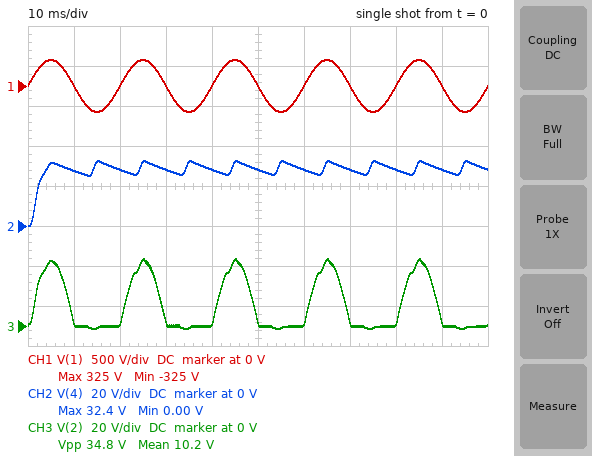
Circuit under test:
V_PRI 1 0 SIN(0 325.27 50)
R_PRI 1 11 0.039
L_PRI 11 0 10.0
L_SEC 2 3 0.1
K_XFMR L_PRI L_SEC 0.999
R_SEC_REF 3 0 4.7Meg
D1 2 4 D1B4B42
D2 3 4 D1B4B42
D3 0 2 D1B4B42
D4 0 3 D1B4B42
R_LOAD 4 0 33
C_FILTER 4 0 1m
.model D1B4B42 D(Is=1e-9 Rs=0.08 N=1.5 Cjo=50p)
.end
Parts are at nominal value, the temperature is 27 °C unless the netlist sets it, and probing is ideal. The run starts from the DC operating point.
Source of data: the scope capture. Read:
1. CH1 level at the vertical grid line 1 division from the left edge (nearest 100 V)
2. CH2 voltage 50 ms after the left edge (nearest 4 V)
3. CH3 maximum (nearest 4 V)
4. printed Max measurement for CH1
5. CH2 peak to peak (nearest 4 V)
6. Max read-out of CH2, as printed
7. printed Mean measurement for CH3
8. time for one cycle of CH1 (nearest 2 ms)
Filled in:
0 V
28 V
32 V
325 V
32 V
32.4 V
10.2 V
20 ms
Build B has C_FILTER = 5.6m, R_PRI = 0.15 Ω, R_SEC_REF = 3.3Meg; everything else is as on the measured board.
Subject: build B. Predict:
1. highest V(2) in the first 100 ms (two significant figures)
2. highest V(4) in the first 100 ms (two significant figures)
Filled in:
35 V
34 V
